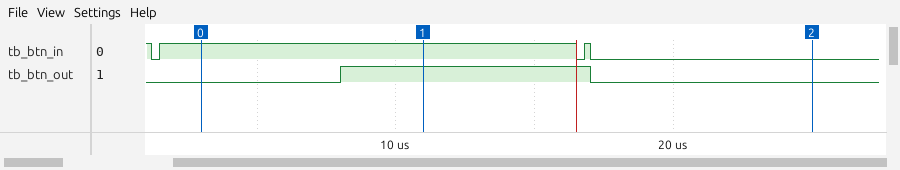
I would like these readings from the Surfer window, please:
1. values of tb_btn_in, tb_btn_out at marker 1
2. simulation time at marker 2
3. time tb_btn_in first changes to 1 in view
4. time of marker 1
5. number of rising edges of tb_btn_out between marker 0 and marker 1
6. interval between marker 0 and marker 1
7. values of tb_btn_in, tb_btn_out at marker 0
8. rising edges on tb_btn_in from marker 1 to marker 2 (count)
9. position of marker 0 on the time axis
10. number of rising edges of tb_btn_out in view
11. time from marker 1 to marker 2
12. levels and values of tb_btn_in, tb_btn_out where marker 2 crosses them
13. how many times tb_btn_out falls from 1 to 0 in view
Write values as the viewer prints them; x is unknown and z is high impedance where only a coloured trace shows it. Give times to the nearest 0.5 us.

tb_btn_in=1, tb_btn_out=1
25 us
1.5 us
11 us
1
8 us
tb_btn_in=1, tb_btn_out=0
1
3 us
1
14 us
tb_btn_in=0, tb_btn_out=0
1
